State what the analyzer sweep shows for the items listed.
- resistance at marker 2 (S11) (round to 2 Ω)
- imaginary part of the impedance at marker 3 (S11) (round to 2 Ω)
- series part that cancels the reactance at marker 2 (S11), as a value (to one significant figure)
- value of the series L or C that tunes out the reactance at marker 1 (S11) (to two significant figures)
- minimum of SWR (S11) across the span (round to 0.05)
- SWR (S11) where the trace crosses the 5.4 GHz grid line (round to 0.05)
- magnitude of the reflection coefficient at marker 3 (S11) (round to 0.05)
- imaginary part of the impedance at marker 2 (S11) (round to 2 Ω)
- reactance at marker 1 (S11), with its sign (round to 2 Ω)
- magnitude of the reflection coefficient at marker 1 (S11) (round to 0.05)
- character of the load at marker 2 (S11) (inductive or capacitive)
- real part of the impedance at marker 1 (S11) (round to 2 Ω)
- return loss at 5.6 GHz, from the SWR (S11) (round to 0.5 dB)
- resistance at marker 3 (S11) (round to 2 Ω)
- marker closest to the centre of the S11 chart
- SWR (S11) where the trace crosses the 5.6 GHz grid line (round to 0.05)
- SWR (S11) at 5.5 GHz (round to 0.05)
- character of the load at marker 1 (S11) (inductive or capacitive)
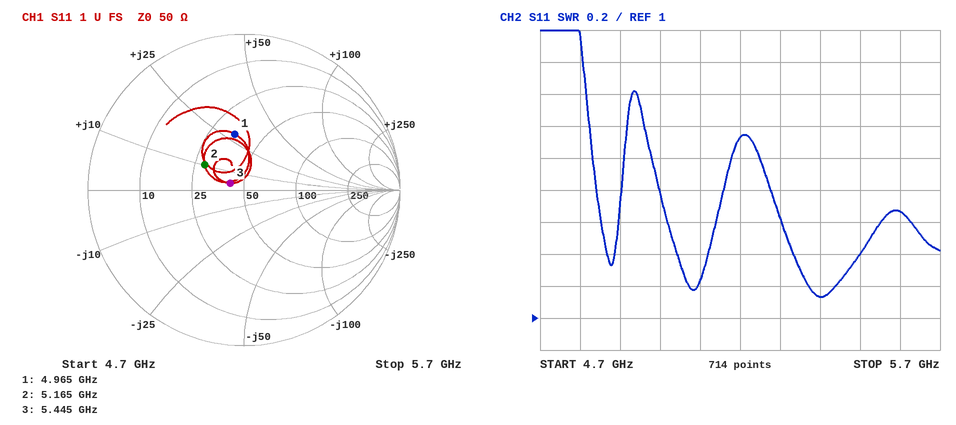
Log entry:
28 Ω
+4 Ω
3 pF
1.1 pF
1.15
1.15
0.10
+10 Ω
+28 Ω
0.35
inductive
34 Ω
12.0 dB
42 Ω
marker 3
1.65
1.40
inductive
